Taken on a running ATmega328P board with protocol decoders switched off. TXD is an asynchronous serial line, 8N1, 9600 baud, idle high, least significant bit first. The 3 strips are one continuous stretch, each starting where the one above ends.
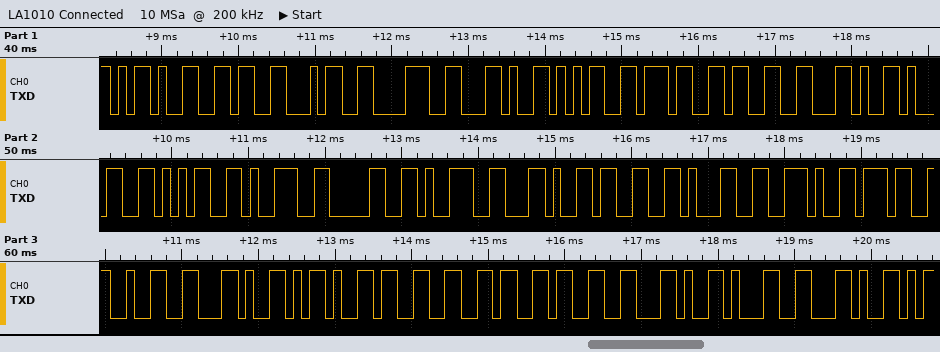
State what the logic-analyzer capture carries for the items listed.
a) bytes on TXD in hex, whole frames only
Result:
0x2D 0x36 0x34 0x38 0x2C 0x35 0x37 0x33 0x2C 0x31 0x35 0x39 0x30 0x39 0x2C 0x33 0x31 0x2E 0x37 0x32 0x2C 0x2D 0x33 0x36 0x33 0x2C 0x31 0x2C
